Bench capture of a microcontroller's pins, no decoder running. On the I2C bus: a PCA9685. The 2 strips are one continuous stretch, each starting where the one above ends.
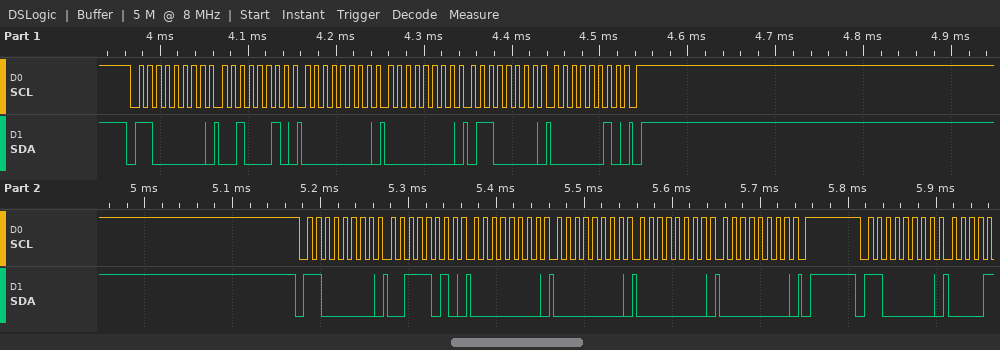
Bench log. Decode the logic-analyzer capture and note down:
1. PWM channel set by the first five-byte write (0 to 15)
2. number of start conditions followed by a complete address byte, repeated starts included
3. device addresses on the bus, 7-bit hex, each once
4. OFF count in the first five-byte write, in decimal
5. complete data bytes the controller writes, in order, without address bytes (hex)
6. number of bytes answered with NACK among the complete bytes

7
3
0x60
608
22 00 00 60 02 3A 00 00 00 00
0
